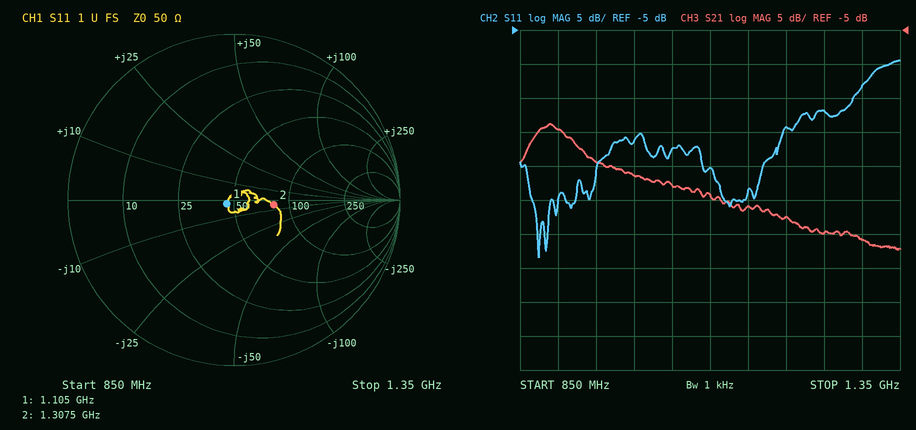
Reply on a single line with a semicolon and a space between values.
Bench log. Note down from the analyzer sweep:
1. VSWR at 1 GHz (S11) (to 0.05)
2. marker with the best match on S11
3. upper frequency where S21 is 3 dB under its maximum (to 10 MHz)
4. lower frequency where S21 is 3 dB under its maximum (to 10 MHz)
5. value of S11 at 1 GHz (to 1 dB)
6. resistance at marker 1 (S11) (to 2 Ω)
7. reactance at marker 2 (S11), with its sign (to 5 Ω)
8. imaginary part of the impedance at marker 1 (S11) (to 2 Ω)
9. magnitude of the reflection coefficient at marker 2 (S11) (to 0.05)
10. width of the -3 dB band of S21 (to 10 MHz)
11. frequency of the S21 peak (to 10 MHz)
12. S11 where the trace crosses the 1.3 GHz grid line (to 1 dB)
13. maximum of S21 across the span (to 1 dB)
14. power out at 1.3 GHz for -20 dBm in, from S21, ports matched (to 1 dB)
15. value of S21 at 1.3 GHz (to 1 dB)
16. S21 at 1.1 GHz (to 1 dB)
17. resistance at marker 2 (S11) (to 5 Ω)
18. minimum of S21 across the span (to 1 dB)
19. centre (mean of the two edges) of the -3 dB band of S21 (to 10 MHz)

1.20; marker 1; 920 MHz; 860 MHz; -21 dB; 46 Ω; -5 Ω; -2 Ω; 0.25; 60 MHz; 890 MHz; -13 dB; -19 dB; -56 dBm; -36 dB; -29 dB; 80 Ω; -37 dB; 890 MHz
